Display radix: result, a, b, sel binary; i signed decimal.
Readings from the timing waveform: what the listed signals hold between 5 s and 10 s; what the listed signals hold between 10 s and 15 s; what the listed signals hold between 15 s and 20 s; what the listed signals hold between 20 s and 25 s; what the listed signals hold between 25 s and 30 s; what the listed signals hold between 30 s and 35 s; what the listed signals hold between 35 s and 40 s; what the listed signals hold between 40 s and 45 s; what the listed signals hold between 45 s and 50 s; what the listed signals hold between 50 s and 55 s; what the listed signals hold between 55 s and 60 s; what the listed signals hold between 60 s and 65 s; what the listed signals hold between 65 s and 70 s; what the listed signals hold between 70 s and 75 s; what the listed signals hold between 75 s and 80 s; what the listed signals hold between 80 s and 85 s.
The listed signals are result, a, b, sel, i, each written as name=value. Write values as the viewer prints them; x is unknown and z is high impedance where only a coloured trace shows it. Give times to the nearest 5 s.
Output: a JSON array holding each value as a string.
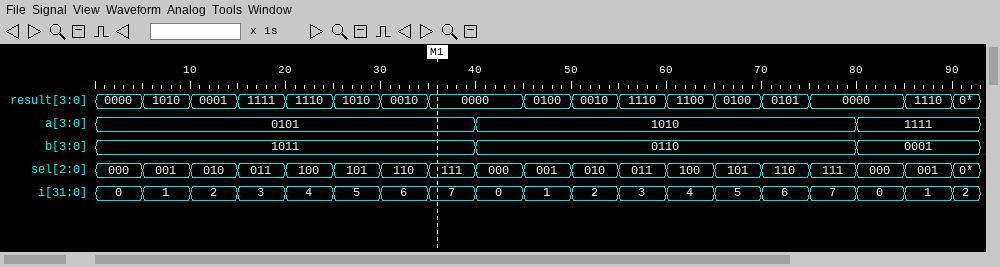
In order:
["result=1010, a=0101, b=1011, sel=001, i=1", "result=0001, a=0101, b=1011, sel=010, i=2", "result=1111, a=0101, b=1011, sel=011, i=3", "result=1110, a=0101, b=1011, sel=100, i=4", "result=1010, a=0101, b=1011, sel=101, i=5", "result=0010, a=0101, b=1011, sel=110, i=6", "result=0000, a=0101, b=1011, sel=111, i=7", "result=0000, a=1010, b=0110, sel=000, i=0", "result=0100, a=1010, b=0110, sel=001, i=1", "result=0010, a=1010, b=0110, sel=010, i=2", "result=1110, a=1010, b=0110, sel=011, i=3", "result=1100, a=1010, b=0110, sel=100, i=4", "result=0100, a=1010, b=0110, sel=101, i=5", "result=0101, a=1010, b=0110, sel=110, i=6", "result=0000, a=1010, b=0110, sel=111, i=7", "result=0000, a=1111, b=0001, sel=000, i=0"]
